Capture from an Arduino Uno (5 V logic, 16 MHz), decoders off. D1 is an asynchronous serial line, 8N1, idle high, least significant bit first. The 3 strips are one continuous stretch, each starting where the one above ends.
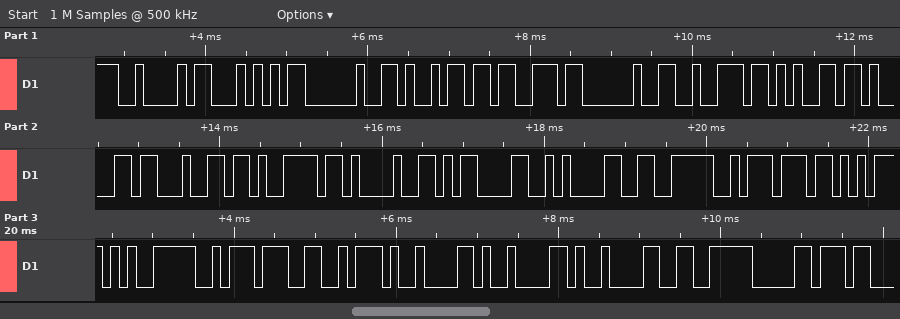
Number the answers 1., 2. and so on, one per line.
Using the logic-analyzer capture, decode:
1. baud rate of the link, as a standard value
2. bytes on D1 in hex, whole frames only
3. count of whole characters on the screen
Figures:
1. 9600 baud
2. 42 54 20 69 73 20 72 65 61 64 79 21 0D 0A E6 BA AB E5 BA A6 09 09 09 E6 B0
3. 25
